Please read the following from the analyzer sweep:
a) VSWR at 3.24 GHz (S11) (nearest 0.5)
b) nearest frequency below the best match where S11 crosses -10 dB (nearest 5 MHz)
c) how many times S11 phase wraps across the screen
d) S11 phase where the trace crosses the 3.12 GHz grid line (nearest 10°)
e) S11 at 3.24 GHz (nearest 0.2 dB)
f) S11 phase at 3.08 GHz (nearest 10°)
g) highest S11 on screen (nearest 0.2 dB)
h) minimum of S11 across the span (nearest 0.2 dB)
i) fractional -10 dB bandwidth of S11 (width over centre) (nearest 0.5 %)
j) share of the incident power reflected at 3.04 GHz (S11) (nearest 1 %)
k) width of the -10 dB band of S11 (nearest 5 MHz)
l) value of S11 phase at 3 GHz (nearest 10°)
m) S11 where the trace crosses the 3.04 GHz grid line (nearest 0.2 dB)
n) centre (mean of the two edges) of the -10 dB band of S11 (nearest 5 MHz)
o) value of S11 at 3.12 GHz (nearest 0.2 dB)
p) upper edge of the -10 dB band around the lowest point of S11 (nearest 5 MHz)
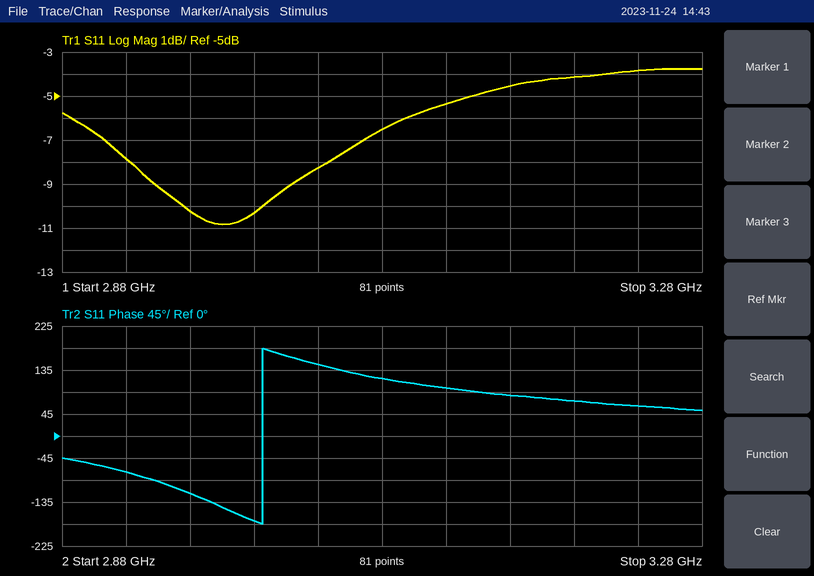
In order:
4.5
2.955 GHz
1
100°
-3.8 dB
120°
-3.8 dB
-10.8 dB
1.5 %
15 %
50 MHz
-170°
-8.2 dB
2.980 GHz
-5.4 dB
3.005 GHz
